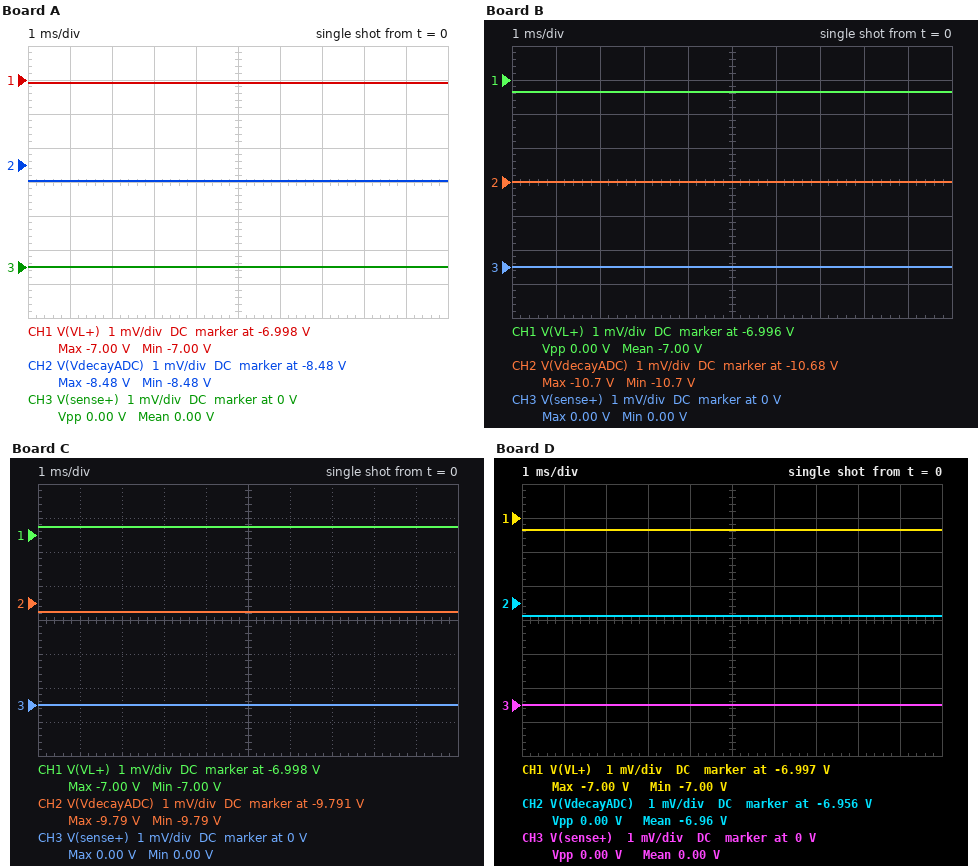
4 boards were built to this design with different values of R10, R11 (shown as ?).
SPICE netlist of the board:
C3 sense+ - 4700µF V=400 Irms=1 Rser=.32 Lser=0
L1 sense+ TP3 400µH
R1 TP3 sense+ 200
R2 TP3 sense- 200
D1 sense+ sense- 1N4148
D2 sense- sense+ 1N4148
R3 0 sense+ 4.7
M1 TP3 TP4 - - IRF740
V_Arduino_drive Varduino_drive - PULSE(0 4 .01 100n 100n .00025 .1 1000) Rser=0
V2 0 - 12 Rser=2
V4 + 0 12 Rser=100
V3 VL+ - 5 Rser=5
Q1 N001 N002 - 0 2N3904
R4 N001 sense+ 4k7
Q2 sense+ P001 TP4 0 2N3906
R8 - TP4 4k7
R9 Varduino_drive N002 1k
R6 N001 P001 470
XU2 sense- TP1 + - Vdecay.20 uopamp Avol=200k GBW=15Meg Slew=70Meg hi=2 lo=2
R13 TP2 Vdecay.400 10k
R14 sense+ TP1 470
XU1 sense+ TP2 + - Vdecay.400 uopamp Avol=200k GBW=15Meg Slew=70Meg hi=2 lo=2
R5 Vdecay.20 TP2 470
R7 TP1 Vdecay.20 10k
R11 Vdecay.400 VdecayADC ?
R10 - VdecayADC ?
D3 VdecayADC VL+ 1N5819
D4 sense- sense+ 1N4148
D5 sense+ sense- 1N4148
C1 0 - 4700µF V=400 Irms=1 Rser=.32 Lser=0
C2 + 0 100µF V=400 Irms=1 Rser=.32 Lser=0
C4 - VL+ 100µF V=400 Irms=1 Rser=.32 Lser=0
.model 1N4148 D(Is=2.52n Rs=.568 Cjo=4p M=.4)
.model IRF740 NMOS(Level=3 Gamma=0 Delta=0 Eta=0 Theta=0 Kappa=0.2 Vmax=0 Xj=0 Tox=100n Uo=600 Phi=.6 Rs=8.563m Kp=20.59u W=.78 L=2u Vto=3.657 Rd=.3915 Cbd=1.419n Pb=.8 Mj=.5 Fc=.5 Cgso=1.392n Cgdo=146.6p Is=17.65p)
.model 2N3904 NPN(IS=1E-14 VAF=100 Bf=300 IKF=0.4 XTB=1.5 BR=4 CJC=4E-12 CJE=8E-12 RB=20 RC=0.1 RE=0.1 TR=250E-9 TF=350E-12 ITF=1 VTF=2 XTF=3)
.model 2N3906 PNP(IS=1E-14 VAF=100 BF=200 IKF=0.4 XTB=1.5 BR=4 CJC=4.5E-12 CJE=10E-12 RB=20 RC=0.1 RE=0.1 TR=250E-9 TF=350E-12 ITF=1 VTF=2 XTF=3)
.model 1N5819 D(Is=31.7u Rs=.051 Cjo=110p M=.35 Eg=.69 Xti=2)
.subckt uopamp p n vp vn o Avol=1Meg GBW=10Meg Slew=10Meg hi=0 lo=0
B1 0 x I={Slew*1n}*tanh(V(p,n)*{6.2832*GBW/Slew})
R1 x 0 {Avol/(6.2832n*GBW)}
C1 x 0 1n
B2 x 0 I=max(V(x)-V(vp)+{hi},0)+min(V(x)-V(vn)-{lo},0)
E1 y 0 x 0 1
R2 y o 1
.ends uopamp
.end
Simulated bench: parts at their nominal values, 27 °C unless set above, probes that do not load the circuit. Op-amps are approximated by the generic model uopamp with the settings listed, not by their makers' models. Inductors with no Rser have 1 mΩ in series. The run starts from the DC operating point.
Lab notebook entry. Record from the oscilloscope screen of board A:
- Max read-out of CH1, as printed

-7.00 V
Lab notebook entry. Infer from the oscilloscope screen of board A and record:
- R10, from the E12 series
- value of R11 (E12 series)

3.3 kΩ
8.2 kΩ
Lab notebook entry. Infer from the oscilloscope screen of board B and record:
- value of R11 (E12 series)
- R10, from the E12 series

5.6 kΩ
680 Ω
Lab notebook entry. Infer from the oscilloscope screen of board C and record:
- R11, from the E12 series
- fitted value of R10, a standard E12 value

8.2 kΩ
1.8 kΩ
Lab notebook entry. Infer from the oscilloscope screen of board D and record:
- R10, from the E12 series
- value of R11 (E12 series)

5.6 kΩ
6.8 kΩ
